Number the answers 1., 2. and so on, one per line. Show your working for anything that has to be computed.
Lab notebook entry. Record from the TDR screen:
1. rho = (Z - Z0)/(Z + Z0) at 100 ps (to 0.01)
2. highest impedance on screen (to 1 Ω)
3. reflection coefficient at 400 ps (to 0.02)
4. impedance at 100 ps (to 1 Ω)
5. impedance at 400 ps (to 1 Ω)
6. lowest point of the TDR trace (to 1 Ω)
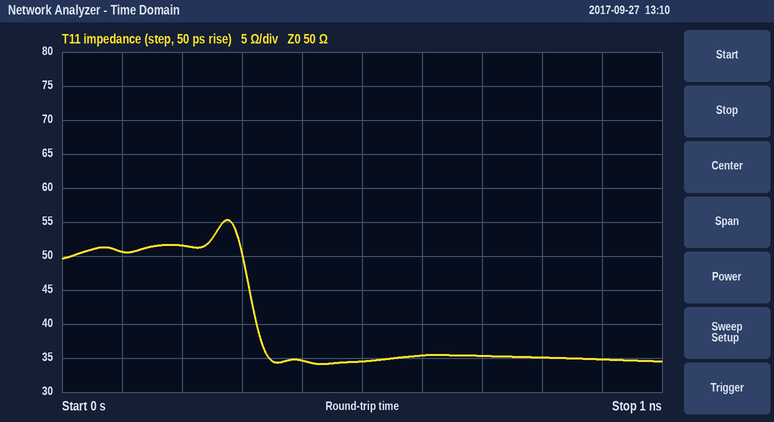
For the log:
1. (51 − 50)/(51 + 50) ≈ +0.01
2. 55 Ω
3. (35 − 50)/(35 + 50) ≈ -0.18
4. 51 Ω
5. 35 Ω
6. 34 Ω
